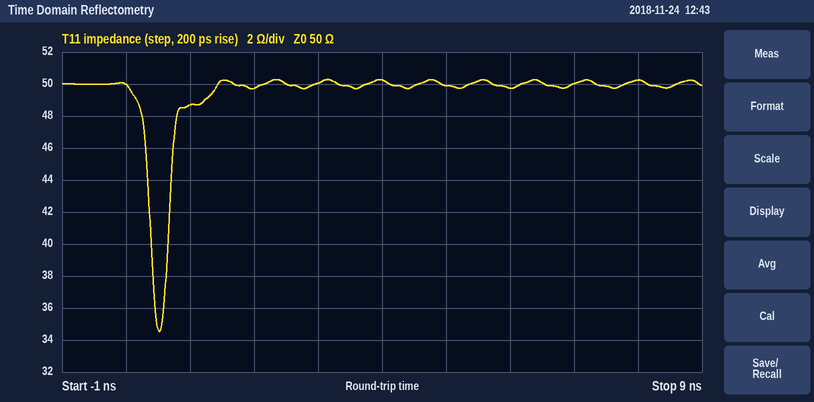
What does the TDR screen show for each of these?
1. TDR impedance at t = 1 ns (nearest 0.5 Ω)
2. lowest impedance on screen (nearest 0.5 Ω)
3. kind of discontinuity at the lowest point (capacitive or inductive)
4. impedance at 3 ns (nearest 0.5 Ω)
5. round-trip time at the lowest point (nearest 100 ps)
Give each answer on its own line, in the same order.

48.5 Ω
34.5 Ω
capacitive
50.0 Ω
500 ps
